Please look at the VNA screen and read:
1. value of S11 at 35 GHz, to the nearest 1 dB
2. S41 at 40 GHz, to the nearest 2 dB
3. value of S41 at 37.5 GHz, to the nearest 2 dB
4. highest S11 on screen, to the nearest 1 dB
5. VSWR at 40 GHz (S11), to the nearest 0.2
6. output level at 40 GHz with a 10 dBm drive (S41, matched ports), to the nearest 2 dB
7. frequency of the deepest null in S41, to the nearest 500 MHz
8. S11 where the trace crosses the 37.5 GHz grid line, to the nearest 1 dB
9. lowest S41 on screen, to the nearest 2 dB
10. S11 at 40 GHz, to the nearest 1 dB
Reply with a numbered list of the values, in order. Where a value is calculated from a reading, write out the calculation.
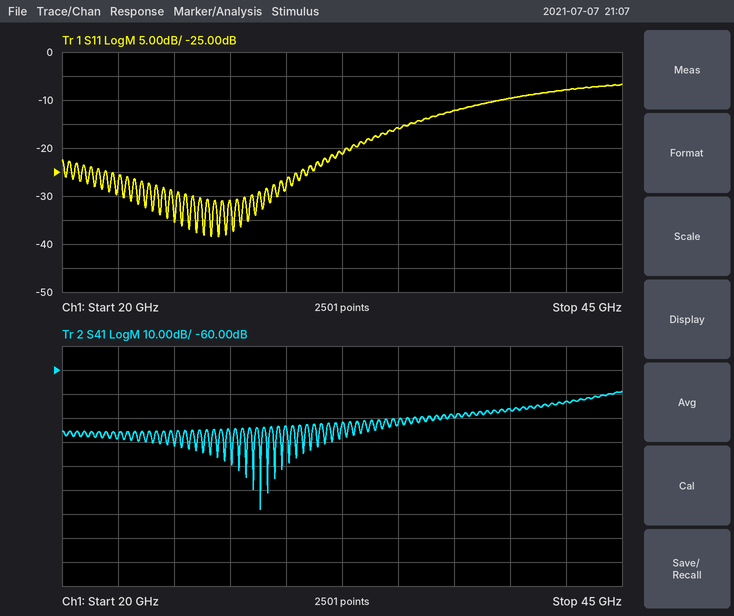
1. -16 dB
2. -76 dB
3. -80 dB
4. -7 dB
5. |Γ| = 10^(-10/20) = 0.3162; VSWR = (1 + 0.3162)/(1 − 0.3162) ≈ 1.92, so 2.0 to the nearest 0.2
6. 10 dBm + (-76 dB) = -66 dBm
7. 29.0 GHz
8. -12 dB
9. -118 dB
10. -10 dB
